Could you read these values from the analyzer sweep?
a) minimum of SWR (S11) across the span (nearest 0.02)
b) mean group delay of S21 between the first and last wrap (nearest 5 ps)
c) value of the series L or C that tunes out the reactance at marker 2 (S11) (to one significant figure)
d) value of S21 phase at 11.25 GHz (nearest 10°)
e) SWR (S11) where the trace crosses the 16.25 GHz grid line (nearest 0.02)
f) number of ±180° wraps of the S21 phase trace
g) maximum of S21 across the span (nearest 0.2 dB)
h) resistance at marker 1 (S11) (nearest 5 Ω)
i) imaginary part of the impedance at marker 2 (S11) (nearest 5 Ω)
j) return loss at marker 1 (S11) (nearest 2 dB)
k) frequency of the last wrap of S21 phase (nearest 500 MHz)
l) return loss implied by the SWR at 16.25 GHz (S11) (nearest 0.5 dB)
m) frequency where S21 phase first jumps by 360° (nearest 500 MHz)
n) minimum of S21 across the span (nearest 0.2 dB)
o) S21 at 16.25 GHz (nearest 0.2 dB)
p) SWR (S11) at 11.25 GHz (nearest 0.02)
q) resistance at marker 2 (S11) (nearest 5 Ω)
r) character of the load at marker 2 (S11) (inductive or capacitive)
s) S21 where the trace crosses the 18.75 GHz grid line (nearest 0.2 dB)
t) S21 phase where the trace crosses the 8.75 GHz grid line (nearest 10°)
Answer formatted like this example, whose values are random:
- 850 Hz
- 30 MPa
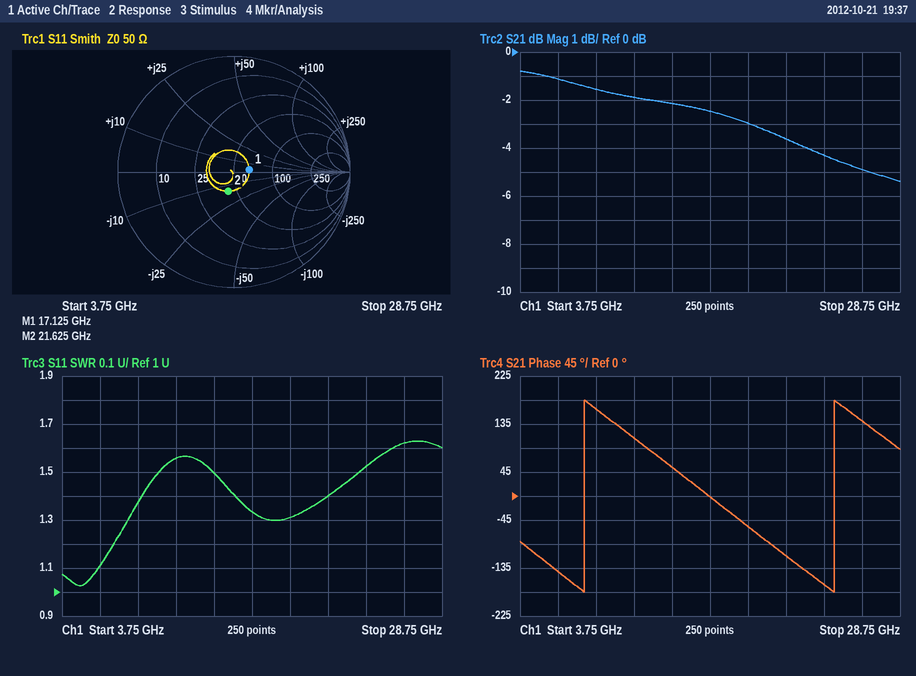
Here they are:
- 1.02
- 60 ps
- 100 pH
- 110°
- 1.34
- 2
- -0.8 dB
- 65 Ω
- -15 Ω
- 18 dB
- 24.5 GHz
- 17.0 dB
- 8.0 GHz
- -5.4 dB
- -2.4 dB
- 1.56
- 45 Ω
- capacitive
- -3.0 dB
- 160°
